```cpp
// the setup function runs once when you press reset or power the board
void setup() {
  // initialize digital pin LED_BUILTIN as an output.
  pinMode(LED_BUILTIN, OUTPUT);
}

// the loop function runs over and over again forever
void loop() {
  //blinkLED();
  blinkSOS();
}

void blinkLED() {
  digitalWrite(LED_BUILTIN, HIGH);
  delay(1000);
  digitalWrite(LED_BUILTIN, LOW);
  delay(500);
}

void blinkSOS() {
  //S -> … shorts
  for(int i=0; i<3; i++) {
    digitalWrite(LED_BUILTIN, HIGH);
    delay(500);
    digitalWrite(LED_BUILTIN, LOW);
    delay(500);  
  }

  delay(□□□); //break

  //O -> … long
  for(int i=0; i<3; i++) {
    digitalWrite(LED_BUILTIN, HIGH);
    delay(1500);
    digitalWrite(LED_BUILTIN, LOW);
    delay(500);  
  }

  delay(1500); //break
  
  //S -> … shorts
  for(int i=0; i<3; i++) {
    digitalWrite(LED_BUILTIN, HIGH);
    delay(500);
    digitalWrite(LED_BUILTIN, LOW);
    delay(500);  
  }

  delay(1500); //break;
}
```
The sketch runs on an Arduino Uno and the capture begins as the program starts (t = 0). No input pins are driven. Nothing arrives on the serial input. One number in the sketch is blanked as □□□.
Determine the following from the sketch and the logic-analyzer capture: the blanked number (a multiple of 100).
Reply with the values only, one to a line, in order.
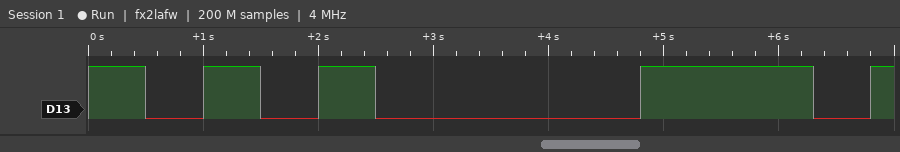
1800
